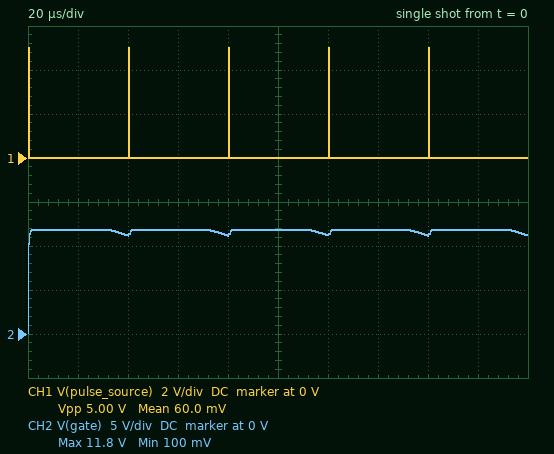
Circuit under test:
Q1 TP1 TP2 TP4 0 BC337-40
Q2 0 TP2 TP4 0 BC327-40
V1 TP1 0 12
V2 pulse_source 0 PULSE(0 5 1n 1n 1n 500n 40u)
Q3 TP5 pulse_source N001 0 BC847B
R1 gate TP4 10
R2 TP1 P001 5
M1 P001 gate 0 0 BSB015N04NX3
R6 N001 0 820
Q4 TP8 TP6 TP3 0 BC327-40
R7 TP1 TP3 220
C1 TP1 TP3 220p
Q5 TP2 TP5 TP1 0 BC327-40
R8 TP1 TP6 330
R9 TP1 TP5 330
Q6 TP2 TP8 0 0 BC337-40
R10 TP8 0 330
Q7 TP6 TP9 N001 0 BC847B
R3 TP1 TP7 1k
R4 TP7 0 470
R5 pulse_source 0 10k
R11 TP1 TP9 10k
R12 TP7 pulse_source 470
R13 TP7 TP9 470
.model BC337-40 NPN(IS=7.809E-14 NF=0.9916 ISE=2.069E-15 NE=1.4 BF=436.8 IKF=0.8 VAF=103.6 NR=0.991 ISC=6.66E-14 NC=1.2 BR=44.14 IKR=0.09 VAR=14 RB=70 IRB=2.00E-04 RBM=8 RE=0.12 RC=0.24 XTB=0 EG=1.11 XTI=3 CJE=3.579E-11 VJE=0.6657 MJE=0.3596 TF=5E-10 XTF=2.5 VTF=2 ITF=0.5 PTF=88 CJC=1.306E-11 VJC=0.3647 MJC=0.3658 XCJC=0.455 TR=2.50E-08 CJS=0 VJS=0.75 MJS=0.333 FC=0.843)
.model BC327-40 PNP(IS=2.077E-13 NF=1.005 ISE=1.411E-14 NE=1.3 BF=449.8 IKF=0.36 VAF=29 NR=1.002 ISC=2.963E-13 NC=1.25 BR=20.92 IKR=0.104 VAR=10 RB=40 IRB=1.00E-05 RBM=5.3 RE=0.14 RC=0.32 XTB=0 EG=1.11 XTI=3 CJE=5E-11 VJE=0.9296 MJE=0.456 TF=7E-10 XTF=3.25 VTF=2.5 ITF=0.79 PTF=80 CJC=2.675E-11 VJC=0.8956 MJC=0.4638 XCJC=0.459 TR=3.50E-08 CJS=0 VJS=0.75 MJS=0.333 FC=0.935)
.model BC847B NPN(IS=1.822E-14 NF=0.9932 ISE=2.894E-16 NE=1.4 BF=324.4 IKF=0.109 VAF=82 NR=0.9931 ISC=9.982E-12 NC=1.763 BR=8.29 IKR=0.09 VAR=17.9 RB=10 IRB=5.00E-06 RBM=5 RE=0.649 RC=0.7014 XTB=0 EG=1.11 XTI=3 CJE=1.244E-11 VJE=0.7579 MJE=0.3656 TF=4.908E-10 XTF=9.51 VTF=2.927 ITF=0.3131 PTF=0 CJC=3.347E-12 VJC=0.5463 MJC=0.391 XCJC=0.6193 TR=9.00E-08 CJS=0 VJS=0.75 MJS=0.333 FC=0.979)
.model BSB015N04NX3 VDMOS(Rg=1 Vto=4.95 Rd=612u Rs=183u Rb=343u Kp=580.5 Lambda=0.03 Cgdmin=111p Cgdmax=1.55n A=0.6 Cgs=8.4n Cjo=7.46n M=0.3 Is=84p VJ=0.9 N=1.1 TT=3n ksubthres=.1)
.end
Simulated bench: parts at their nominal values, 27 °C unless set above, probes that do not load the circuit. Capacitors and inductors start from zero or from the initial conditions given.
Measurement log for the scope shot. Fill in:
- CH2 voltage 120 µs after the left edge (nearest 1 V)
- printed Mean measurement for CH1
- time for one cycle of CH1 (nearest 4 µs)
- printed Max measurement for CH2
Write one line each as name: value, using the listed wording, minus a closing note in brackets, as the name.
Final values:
CH2 voltage 120 µs after the left edge: 11 V
printed Mean measurement for CH1: 60.0 mV
time for one cycle of CH1: 40 µs
printed Max measurement for CH2: 11.8 V
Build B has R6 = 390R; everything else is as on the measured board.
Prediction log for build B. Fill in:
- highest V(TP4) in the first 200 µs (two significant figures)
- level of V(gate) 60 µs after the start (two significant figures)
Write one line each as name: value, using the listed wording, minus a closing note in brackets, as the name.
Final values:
highest V(TP4) in the first 200 µs: 11 V
level of V(gate) 60 µs after the start: 470 mV
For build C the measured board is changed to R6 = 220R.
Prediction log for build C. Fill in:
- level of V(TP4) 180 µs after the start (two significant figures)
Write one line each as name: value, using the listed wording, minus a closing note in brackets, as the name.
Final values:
level of V(TP4) 180 µs after the start: 470 mV
